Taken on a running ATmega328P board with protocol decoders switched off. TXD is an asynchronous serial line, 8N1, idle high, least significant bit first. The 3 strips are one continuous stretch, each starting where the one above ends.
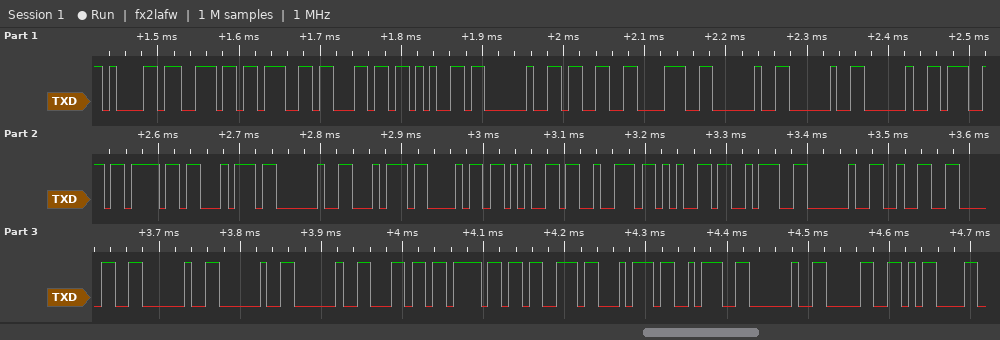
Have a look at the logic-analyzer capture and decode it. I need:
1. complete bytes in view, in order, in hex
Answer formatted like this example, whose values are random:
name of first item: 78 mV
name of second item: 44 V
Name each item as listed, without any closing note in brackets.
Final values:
complete bytes in view, in order, in hex: 61 6E 67 6C 65 20 33 38 20 20 20 67 6F 74 20 74 68 65 72 65 3A 20 32 30 20 20 20 6C 6F 73 74 3A 20 30 0D
